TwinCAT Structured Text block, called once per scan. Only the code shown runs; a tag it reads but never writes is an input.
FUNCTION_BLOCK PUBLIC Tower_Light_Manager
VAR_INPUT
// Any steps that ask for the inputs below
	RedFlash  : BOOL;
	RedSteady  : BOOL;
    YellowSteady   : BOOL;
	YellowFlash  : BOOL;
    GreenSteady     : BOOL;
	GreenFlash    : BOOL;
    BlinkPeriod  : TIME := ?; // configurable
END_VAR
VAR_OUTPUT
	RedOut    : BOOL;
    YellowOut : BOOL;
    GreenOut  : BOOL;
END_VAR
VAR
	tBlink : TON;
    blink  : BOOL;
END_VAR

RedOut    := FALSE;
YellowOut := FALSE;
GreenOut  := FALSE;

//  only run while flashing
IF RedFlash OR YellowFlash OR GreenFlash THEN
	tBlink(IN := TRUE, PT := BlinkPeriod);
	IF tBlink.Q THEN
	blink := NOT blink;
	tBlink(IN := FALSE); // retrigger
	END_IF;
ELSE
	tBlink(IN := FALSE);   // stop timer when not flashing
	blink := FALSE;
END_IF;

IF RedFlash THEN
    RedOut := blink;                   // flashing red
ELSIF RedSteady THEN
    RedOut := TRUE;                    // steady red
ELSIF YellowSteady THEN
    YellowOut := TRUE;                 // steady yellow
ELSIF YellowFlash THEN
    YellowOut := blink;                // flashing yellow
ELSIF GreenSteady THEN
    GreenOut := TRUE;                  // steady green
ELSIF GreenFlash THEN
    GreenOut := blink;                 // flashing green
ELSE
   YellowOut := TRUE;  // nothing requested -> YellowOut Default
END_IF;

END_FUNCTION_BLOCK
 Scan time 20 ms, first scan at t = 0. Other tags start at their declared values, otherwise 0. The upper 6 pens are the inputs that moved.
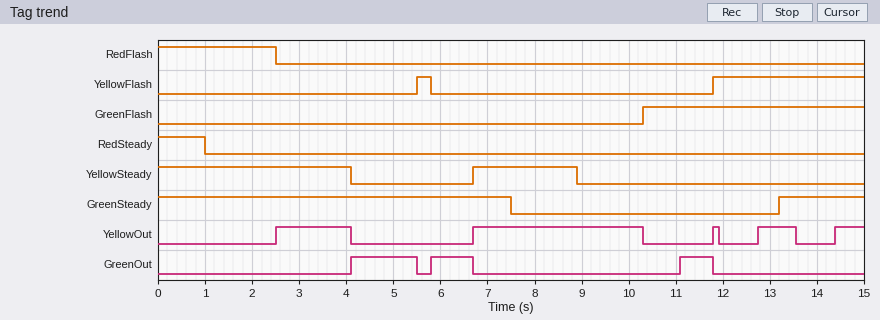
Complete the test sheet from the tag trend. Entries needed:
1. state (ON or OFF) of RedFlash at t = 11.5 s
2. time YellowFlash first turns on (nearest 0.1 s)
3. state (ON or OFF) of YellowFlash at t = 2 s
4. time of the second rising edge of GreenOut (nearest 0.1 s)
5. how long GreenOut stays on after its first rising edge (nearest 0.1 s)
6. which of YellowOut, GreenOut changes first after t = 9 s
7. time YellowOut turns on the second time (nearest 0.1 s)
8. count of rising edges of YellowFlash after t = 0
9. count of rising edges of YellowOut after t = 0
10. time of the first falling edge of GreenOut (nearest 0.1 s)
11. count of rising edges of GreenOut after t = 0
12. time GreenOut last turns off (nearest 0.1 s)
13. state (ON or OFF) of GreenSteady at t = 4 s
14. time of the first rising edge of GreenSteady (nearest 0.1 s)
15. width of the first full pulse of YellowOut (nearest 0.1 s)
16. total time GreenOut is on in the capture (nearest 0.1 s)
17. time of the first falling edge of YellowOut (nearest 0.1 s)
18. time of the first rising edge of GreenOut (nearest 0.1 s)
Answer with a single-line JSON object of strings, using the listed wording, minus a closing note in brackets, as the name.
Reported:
{"state (ON or OFF) of RedFlash at t = 11.5 s": "OFF", "time YellowFlash first turns on": "5.5 s", "state (ON or OFF) of YellowFlash at t = 2 s": "OFF", "time of the second rising edge of GreenOut": "5.8 s", "how long GreenOut stays on after its first rising edge": "1.4 s", "which of YellowOut, GreenOut changes first after t = 9 s": "YellowOut", "time YellowOut turns on the second time": "6.7 s", "count of rising edges of YellowFlash after t = 0": "2", "count of rising edges of YellowOut after t = 0": "5", "time of the first falling edge of GreenOut": "5.5 s", "count of rising edges of GreenOut after t = 0": "3", "time GreenOut last turns off": "11.8 s", "state (ON or OFF) of GreenSteady at t = 4 s": "ON", "time of the first rising edge of GreenSteady": "13.2 s", "width of the first full pulse of YellowOut": "1.6 s", "total time GreenOut is on in the capture": "3.0 s", "time of the first falling edge of YellowOut": "4.1 s", "time of the first rising edge of GreenOut": "4.1 s"}
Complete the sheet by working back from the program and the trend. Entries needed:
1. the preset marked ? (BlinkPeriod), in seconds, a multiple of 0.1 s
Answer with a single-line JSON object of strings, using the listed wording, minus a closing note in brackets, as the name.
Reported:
{"the preset marked ? (BlinkPeriod), in seconds, a multiple of 0.1 s": "0.8 s"}
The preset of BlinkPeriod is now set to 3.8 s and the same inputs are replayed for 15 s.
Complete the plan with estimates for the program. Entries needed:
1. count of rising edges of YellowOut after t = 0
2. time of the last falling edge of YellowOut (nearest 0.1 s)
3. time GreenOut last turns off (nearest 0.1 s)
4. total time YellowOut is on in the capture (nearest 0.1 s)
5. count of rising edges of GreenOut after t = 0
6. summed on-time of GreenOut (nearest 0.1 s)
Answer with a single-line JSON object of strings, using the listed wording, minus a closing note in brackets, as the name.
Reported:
{"count of rising edges of YellowOut after t = 0": "3", "time of the last falling edge of YellowOut": "10.3 s", "time GreenOut last turns off": "6.7 s", "total time YellowOut is on in the capture": "6.1 s", "count of rising edges of GreenOut after t = 0": "2", "summed on-time of GreenOut": "2.3 s"}
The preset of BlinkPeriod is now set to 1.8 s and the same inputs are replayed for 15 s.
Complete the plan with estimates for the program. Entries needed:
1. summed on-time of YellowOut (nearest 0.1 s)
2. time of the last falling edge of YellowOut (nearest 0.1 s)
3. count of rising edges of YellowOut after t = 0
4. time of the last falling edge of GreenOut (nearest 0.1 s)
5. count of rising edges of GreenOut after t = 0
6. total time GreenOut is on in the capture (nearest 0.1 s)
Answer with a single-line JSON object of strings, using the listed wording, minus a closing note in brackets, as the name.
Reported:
{"summed on-time of YellowOut": "7.0 s", "time of the last falling edge of YellowOut": "13.9 s", "count of rising edges of YellowOut after t = 0": "3", "time of the last falling edge of GreenOut": "6.7 s", "count of rising edges of GreenOut after t = 0": "2", "total time GreenOut is on in the capture": "2.3 s"}
